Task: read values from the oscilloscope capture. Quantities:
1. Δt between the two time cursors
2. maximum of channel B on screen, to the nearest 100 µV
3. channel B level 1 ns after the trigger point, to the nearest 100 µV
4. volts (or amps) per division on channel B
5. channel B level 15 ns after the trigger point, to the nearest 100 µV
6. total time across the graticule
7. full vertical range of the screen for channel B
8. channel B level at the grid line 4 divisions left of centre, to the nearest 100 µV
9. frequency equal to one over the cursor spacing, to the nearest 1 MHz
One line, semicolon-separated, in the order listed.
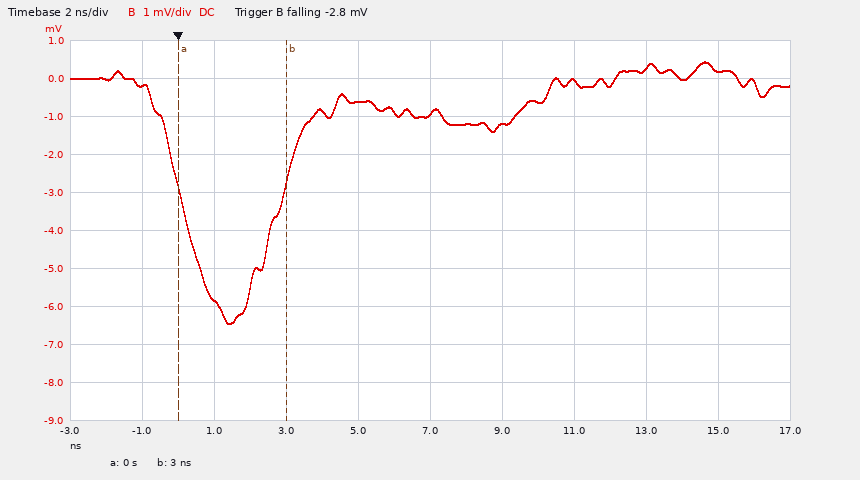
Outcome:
3.0 ns; 400 µV; -5.8 mV; 1 mV; 200 µV; 20 ns; 10 mV; -200 µV; 333 MHz
